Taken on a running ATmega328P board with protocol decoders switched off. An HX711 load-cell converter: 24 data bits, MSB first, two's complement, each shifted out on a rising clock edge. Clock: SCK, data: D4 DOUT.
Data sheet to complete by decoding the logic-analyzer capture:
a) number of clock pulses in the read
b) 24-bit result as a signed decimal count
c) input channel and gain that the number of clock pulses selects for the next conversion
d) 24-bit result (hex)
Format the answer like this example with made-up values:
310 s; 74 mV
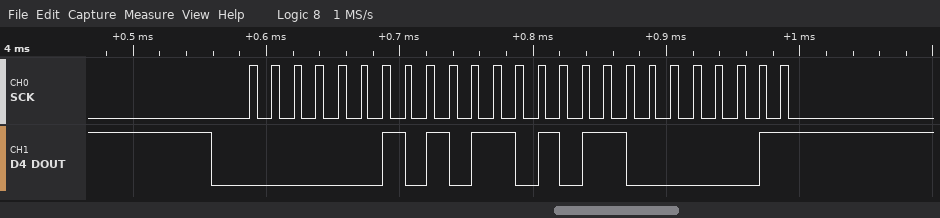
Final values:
25; 177537; channel A, gain 128; 0x02B581
